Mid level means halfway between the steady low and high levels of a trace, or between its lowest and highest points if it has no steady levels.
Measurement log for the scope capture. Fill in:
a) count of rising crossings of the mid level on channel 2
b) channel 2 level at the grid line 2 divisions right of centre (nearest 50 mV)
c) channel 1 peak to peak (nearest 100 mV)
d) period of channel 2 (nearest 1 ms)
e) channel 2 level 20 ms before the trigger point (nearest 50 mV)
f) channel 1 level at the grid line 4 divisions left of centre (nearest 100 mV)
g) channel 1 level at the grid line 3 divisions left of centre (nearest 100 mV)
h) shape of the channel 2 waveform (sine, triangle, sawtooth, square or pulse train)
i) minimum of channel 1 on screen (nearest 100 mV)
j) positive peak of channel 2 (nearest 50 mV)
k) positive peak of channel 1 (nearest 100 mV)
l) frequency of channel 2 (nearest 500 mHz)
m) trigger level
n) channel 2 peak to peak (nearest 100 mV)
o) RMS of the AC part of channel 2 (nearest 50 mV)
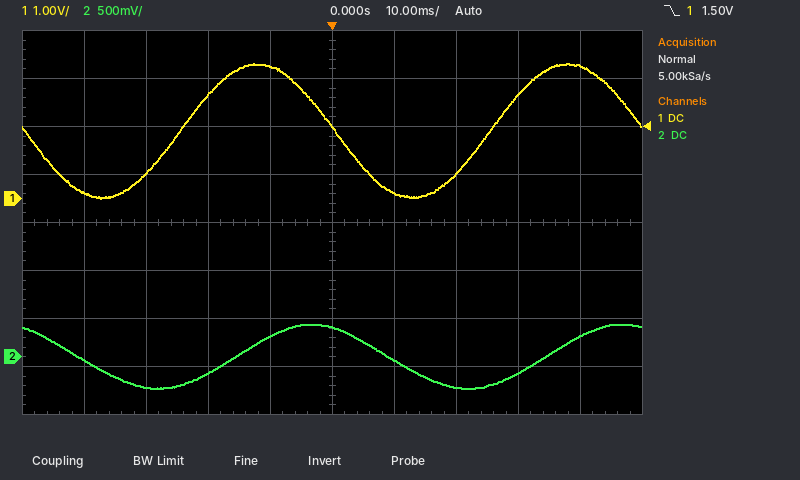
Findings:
2
-300 mV
2.8 V
50 ms
-150 mV
100 mV
500 mV
sine
0.0 V
350 mV
2.8 V
20.0 Hz
1.50 V
700 mV
250 mV
